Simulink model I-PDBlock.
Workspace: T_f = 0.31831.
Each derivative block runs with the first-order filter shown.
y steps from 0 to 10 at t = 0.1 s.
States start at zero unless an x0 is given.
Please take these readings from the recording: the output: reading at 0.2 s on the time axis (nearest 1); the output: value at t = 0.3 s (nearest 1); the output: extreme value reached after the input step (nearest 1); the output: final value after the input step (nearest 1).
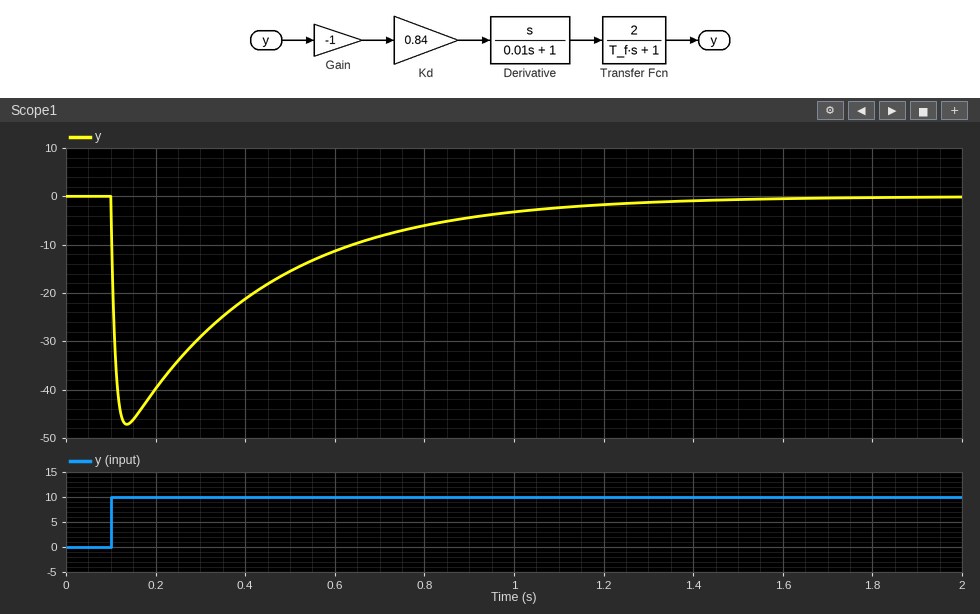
-40
-29
-47
0
